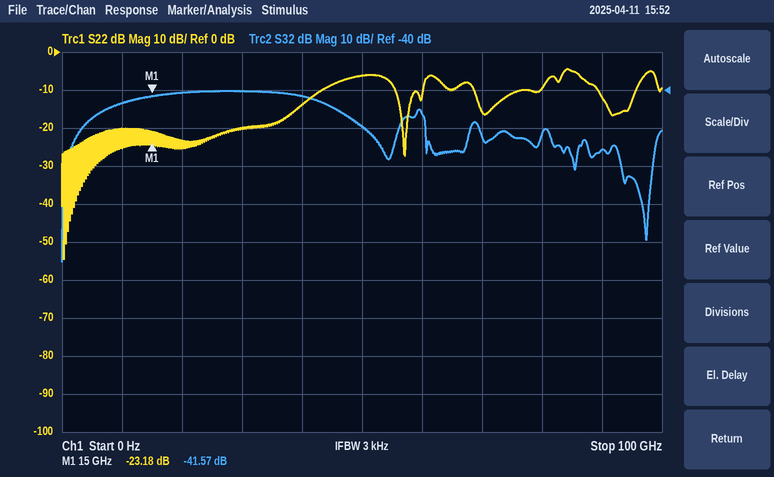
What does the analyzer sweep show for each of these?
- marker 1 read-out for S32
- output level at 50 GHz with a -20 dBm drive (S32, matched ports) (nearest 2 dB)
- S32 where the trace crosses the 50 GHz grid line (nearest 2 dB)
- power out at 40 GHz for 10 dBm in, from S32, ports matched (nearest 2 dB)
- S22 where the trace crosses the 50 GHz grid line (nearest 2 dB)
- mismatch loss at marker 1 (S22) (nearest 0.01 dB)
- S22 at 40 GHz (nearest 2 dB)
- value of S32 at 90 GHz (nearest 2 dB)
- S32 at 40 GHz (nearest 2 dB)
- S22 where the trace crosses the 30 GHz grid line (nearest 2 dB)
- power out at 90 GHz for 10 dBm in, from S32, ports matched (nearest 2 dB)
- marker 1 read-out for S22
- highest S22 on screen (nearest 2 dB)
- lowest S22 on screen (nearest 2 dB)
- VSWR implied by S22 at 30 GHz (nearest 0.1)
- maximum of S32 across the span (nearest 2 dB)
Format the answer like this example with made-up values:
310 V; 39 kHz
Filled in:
-41.57 dB; -70 dBm; -50 dB; -32 dBm; -6 dB; 0.02 dB; -14 dB; -56 dB; -42 dB; -20 dB; -46 dBm; -23.18 dB; -4 dB; -54 dB; 1.2; -40 dB
